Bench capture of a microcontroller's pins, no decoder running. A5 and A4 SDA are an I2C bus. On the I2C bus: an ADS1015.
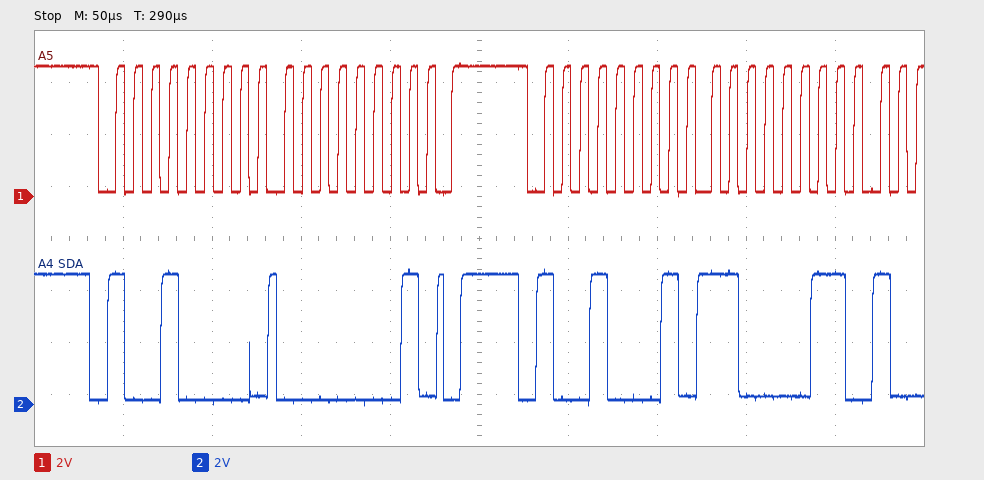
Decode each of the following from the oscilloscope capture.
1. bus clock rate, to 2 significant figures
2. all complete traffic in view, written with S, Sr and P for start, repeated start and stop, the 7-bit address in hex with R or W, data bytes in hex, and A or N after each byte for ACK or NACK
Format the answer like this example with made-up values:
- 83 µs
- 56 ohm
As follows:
- 100 kHz
- S 48W A 01 A P S 48R A C3 A
